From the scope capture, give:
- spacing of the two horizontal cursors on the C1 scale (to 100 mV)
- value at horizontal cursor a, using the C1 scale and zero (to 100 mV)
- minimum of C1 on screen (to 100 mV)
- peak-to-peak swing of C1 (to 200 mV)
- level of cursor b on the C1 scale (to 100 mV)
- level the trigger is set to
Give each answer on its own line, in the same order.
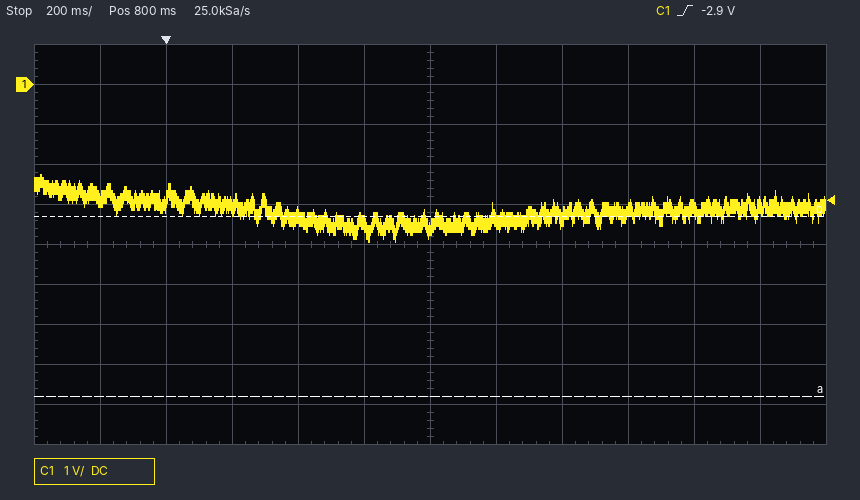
4.5 V
-7.8 V
-3.9 V
1.6 V
-3.3 V
-2.9 V
